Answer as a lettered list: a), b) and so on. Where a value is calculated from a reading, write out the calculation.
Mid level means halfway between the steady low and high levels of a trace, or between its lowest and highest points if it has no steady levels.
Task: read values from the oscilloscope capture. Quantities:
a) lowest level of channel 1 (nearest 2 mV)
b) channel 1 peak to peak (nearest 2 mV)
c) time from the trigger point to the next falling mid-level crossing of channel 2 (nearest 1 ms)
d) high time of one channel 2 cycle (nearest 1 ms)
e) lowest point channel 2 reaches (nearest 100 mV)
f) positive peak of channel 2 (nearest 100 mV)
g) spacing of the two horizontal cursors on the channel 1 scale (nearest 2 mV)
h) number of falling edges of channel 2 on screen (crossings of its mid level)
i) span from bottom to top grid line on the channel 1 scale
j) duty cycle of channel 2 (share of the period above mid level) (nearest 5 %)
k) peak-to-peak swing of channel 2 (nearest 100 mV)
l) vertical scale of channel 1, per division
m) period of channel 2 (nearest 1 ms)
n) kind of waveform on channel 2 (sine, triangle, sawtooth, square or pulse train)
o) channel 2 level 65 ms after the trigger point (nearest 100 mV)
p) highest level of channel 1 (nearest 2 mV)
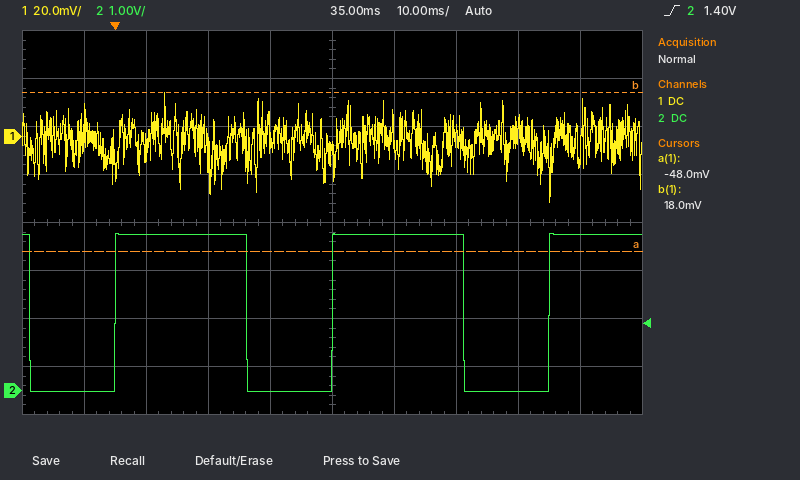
a) -28 mV
b) 18 mV − (-28 mV) = 46 mV
c) 21 ms
d) 21 ms
e) 0.0 V
f) 3.3 V
g) 66 mV
h) 3
i) 160 mV
j) 21 ms / 35 ms ≈ 60 %
k) 3.3 V − (0.0 V) = 3.3 V
l) 20 mV
m) 35 ms
n) pulse train
o) 0.0 V
p) 18 mV
